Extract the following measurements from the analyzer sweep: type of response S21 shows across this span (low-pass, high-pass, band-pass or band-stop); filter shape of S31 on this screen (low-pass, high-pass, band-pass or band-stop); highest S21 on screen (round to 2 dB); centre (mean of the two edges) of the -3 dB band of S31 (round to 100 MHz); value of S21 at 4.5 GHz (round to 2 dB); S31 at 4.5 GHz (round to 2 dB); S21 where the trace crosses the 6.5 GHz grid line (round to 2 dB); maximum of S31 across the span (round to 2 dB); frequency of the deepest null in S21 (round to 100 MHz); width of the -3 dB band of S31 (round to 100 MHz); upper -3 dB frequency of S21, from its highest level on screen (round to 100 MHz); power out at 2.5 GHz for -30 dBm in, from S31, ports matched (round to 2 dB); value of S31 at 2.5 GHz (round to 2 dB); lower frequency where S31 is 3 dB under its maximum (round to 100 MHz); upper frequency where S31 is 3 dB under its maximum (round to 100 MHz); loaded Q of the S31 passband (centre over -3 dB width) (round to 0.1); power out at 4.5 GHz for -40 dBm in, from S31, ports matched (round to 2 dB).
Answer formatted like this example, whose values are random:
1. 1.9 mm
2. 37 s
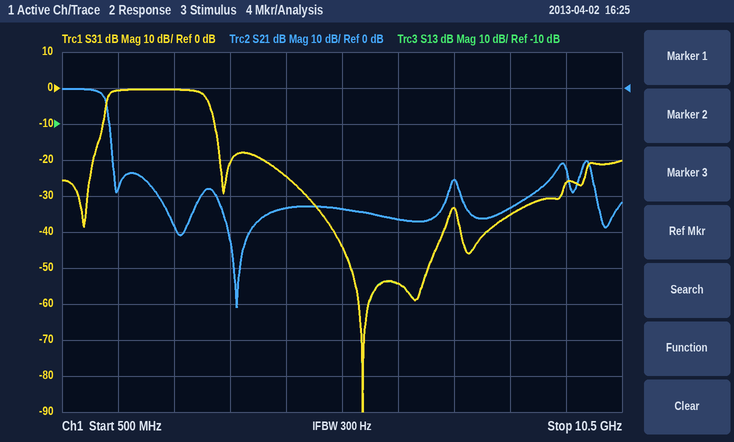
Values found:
1. low-pass
2. band-pass
3. 0 dB
4. 2.2 GHz
5. -34 dB
6. -24 dB
7. -36 dB
8. 0 dB
9. 3.6 GHz
10. 1.8 GHz
11. 1.3 GHz
12. -30 dBm
13. 0 dB
14. 1.3 GHz
15. 3.1 GHz
16. 1.2
17. -64 dBm
